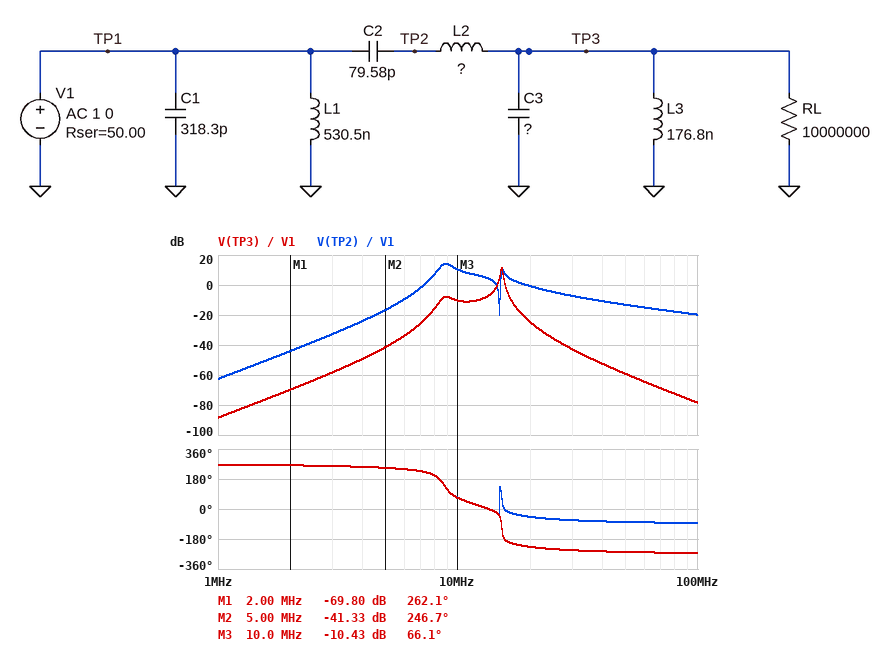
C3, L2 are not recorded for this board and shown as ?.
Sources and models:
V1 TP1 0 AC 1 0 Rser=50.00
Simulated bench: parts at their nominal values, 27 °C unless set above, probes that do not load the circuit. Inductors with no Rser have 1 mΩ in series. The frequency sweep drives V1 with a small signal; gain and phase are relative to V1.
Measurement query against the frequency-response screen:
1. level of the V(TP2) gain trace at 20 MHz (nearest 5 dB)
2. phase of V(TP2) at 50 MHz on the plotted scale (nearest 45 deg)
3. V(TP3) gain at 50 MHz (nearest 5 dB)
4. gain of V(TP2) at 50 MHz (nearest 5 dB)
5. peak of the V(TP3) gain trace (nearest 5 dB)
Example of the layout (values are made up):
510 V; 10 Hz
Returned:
0 dB; -90 deg; -60 dB; -15 dB; 10 dB
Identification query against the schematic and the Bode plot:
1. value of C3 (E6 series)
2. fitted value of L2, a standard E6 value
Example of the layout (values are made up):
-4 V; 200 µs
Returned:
680 pF; 3.3 µH
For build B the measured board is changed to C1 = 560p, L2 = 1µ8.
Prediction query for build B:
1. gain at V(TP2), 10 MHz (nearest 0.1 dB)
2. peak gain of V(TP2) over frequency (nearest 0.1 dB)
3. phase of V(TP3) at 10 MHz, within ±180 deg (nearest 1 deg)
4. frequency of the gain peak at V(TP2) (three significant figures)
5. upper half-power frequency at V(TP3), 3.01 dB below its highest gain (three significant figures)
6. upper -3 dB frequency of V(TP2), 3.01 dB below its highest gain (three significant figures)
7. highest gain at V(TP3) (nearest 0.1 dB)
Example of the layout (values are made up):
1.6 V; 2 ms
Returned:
3.1 dB; 16.1 dB; 134 deg; 16.9 MHz; 17.1 MHz; 17.2 MHz; 7.8 dB
